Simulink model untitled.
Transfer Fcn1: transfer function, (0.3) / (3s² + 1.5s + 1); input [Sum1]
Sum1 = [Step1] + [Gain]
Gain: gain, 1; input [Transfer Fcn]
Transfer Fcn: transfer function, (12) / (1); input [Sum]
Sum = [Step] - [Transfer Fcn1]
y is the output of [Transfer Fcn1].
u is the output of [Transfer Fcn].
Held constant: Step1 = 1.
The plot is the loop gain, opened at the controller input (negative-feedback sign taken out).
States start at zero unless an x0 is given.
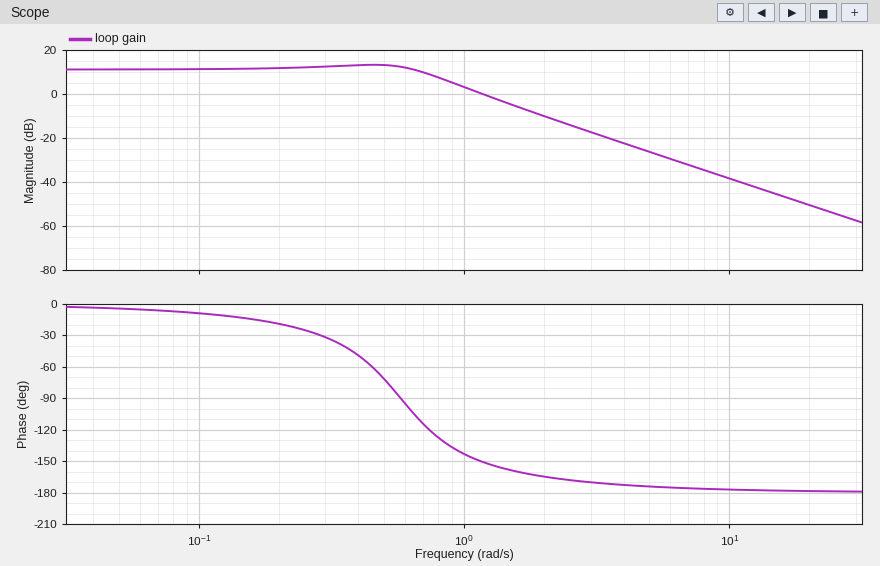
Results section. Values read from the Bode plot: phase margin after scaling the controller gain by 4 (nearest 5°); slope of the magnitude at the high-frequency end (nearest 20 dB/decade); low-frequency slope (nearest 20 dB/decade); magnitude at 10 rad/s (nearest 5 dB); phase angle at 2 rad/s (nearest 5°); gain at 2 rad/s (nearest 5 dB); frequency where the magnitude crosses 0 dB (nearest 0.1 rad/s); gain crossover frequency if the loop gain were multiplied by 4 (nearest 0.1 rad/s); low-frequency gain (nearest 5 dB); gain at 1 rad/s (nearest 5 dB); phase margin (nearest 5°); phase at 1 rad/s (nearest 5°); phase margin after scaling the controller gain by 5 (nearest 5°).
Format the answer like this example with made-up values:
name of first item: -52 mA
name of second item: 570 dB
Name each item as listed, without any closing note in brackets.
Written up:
phase margin after scaling the controller gain by 4: 15°
slope of the magnitude at the high-frequency end: -40 dB/decade
low-frequency slope: 0 dB/decade
magnitude at 10 rad/s: -40 dB
phase angle at 2 rad/s: -165°
gain at 2 rad/s: -10 dB
frequency where the magnitude crosses 0 dB: 1.2 rad/s
gain crossover frequency if the loop gain were multiplied by 4: 2.2 rad/s
low-frequency gain: 10 dB
gain at 1 rad/s: 5 dB
phase margin: 30°
phase at 1 rad/s: -145°
phase margin after scaling the controller gain by 5: 10°
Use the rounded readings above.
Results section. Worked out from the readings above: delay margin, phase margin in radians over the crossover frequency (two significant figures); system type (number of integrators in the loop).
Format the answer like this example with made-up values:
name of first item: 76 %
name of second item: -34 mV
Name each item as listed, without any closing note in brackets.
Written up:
delay margin, phase margin in radians over the crossover frequency: 0.44 s
system type: 0
